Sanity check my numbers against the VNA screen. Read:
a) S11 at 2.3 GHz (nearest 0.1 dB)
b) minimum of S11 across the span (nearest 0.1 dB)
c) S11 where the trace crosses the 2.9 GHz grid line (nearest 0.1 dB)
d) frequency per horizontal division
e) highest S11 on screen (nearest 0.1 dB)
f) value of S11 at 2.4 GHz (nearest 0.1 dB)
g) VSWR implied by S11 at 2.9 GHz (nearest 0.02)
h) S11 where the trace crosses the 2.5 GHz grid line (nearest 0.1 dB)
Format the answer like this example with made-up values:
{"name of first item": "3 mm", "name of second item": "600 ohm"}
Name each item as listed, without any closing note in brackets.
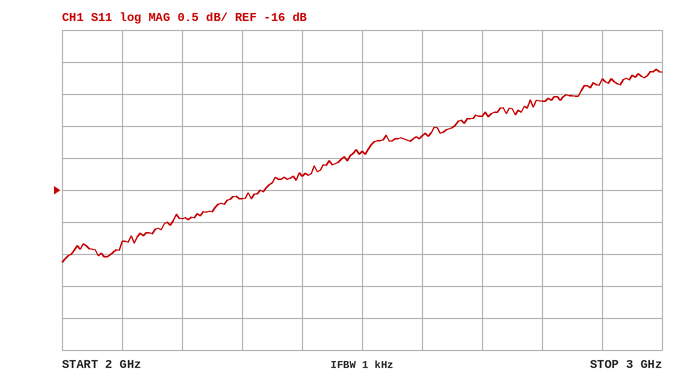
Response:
{"S11 at 2.3 GHz": "-16.1 dB", "minimum of S11 across the span": "-17.1 dB", "S11 where the trace crosses the 2.9 GHz grid line": "-14.3 dB", "frequency per horizontal division": "100 MHz", "highest S11 on screen": "-14.1 dB", "value of S11 at 2.4 GHz": "-15.8 dB", "VSWR implied by S11 at 2.9 GHz": "1.48", "S11 where the trace crosses the 2.5 GHz grid line": "-15.4 dB"}
